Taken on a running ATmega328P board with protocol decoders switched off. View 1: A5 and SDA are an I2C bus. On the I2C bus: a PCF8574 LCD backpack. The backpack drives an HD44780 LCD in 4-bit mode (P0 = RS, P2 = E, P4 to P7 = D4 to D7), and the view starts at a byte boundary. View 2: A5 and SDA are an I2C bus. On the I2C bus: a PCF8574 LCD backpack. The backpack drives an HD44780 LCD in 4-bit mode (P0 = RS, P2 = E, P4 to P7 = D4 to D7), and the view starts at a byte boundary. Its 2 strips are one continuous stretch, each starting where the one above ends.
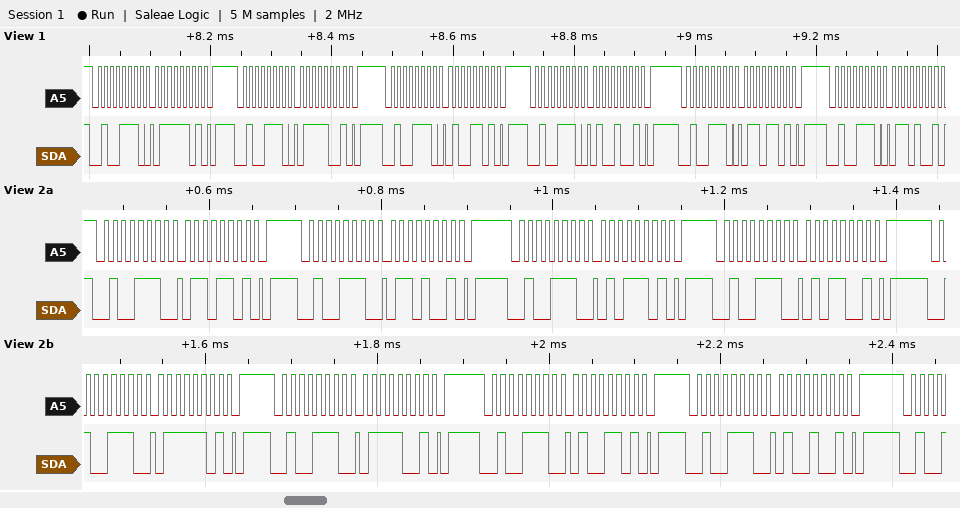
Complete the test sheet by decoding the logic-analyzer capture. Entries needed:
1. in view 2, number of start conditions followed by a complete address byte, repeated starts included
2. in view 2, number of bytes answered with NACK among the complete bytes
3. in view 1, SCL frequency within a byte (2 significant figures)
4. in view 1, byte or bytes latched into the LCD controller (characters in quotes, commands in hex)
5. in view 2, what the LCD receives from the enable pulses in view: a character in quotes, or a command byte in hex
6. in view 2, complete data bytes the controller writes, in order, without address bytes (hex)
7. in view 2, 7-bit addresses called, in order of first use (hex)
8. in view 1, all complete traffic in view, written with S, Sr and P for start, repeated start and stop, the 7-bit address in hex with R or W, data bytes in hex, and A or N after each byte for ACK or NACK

8
0
100 kHz
't'
'e' 't'
6D 69 5D 59 7D 79 4D 49
0x27
S 27W A 7D A P S 27W A 79 A P S 27W A 4D A P S 27W A 49 A P S 27W A 6D A P S 27W A 69 A
